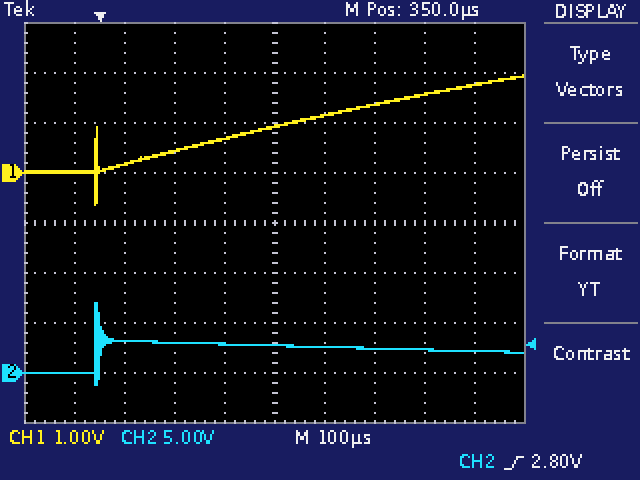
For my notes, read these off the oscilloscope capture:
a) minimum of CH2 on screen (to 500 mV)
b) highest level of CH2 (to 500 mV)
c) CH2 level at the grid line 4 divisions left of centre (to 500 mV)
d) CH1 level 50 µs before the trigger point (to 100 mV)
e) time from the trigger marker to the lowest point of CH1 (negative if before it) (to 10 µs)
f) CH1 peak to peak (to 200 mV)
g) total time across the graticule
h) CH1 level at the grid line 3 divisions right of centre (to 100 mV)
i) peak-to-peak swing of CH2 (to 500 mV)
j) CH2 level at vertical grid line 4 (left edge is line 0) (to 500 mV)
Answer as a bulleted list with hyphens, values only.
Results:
- -1.0 V
- 7.0 V
- 0.0 V
- 0.0 V
- -10 µs
- 2.6 V
- 1 ms
- 1.6 V
- 8.0 V
- 3.0 V
